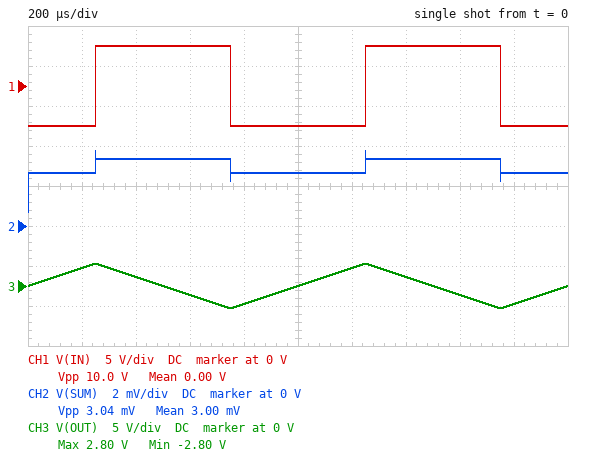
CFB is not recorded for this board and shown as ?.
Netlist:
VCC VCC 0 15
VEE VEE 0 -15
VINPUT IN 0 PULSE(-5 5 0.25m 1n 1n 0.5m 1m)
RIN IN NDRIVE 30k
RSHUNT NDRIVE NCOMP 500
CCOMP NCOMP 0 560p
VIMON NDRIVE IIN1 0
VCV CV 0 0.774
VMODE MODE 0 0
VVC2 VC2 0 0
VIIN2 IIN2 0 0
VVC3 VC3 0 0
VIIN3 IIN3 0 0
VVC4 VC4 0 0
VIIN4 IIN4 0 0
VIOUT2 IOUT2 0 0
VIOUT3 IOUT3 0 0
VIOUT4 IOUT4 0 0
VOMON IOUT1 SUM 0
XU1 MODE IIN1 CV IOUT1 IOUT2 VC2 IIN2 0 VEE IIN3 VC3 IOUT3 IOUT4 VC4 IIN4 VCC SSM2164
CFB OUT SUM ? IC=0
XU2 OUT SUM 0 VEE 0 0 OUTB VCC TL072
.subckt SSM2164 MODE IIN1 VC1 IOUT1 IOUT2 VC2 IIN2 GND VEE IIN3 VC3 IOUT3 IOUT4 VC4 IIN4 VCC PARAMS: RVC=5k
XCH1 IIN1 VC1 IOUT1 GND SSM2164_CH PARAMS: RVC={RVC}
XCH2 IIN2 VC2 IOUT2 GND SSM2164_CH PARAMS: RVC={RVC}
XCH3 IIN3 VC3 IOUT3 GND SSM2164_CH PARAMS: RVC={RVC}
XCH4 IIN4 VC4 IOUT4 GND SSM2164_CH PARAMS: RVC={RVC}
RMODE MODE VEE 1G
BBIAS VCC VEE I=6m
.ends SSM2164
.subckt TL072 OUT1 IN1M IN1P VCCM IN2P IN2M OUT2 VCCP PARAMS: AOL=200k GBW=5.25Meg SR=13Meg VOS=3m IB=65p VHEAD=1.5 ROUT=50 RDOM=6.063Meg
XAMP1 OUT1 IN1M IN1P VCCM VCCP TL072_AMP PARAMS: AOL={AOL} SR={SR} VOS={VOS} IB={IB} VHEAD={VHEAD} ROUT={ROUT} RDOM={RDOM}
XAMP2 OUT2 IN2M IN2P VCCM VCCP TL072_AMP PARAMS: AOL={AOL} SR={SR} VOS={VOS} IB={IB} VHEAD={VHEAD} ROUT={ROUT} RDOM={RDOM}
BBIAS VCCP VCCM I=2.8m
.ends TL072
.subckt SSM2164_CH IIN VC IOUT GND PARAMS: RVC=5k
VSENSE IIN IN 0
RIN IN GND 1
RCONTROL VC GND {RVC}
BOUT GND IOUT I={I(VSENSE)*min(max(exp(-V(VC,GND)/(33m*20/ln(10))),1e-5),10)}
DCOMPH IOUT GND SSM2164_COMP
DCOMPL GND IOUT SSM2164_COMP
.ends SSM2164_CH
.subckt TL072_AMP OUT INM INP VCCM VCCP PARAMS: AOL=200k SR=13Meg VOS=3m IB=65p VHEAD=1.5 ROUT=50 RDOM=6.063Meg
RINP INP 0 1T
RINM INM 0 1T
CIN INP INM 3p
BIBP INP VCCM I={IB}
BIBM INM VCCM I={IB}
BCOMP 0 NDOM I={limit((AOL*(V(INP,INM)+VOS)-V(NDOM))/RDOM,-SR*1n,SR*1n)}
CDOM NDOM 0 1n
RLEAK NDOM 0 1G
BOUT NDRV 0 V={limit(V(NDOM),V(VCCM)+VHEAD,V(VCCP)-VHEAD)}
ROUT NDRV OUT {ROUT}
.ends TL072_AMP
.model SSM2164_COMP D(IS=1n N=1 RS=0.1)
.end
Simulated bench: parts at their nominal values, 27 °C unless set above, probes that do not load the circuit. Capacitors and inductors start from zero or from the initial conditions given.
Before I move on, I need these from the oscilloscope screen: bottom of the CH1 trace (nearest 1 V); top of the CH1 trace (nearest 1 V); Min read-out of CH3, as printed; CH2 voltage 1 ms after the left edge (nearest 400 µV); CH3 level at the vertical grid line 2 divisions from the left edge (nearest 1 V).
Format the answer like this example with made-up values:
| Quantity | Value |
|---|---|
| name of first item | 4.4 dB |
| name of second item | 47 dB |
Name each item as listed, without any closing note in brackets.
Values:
| Quantity | Value |
|---|---|
| bottom of the CH1 trace | -5 V |
| top of the CH1 trace | 5 V |
| Min read-out of CH3, as printed | -2.80 V |
| CH2 voltage 1 ms after the left edge | 2.8 mV |
| CH3 level at the vertical grid line 2 divisions from the left edge | 1 V |
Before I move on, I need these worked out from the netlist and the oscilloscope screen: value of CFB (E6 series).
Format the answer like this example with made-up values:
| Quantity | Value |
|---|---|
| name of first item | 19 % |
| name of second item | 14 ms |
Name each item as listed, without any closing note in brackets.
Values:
| Quantity | Value |
|---|---|
| value of CFB | 1 nF |
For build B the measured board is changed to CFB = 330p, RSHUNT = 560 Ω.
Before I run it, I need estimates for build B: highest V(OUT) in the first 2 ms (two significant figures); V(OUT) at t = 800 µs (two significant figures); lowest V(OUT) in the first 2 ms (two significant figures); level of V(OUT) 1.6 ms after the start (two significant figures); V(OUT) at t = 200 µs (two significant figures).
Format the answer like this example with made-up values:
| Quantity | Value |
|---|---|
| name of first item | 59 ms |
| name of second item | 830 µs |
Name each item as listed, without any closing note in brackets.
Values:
| Quantity | Value |
|---|---|
| highest V(OUT) in the first 2 ms | 8.5 V |
| V(OUT) at t = 800 µs | -6.8 V |
| lowest V(OUT) in the first 2 ms | -8.5 V |
| level of V(OUT) 1.6 ms after the start | -3.4 V |
| V(OUT) at t = 200 µs | 6.8 V |
